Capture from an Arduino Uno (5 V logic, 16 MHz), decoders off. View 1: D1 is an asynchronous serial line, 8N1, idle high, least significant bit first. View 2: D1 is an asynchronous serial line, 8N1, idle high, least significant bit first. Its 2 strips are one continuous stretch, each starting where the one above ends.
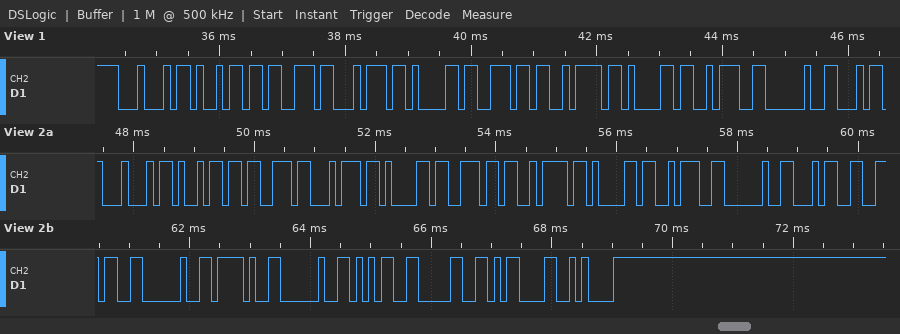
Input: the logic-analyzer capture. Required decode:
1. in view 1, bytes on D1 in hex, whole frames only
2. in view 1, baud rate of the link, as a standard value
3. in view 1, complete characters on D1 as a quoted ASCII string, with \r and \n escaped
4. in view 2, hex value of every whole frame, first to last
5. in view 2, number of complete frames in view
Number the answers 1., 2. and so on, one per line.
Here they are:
1. 44 69 73 74 61 6E 7A 61 3A 20
2. 9600 baud
3. "Distanza: "
4. 44 69 73 74 61 6E 7A 61 3A 20 34 36 20 2F 20 35 30 0D 0A
5. 19
